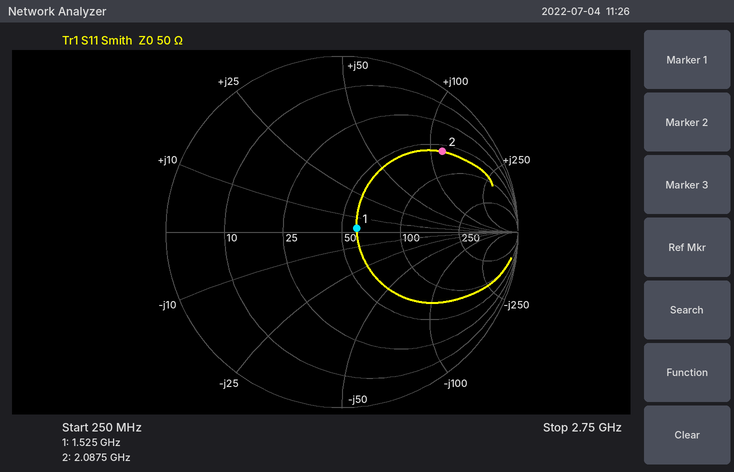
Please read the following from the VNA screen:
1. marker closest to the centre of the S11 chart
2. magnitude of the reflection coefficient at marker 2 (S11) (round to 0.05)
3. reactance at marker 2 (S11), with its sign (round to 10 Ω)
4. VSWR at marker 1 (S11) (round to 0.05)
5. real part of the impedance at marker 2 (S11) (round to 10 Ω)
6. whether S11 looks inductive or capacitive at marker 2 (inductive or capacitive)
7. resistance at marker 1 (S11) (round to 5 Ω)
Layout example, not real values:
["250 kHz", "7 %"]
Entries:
["marker 1", "0.75", "+120 Ω", "1.20", "60 Ω", "inductive", "60 Ω"]
